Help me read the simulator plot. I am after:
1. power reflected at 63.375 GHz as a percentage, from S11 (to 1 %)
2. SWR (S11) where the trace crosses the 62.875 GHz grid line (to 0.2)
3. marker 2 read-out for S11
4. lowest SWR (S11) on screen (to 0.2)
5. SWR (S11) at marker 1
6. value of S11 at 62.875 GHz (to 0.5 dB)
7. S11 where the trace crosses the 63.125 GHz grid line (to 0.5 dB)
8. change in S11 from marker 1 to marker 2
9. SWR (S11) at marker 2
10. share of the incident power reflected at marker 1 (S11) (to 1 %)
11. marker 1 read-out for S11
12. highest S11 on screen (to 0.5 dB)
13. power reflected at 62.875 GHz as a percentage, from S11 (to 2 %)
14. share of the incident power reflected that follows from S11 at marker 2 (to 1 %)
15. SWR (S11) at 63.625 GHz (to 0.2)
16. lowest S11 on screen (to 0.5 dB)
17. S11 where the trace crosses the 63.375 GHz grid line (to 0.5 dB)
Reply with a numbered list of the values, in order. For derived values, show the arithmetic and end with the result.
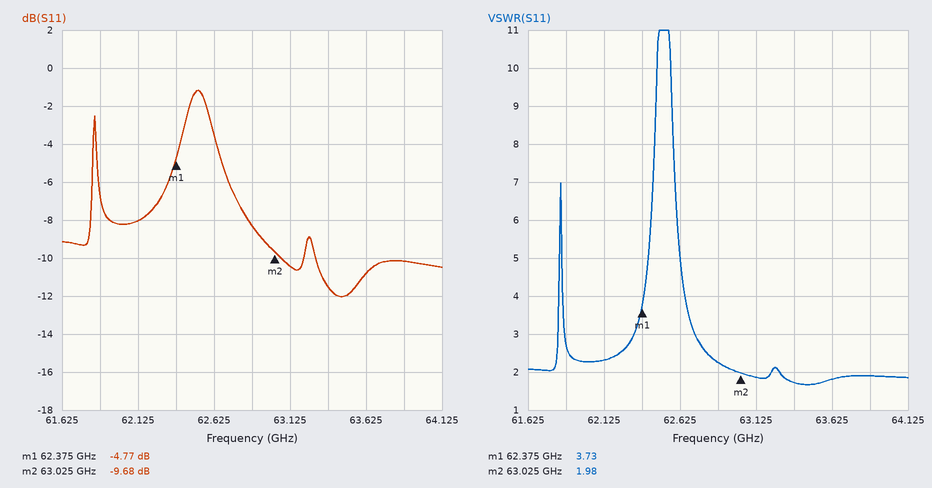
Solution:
1. 10^(-11.5/10) ≈ 7 %
2. 2.2
3. -9.68 dB
4. 1.6
5. 3.73
6. -8.5 dB
7. -10.5 dB
8. -9.68 − (-4.77) = -4.91 dB
9. 1.98
10. 10^(-4.77/10) ≈ 33 %
11. -4.77 dB
12. -1.0 dB
13. 10^(-8.5/10) ≈ 14 %
14. 10^(-9.68/10) ≈ 11 %
15. 1.8
16. -12.0 dB
17. -11.5 dB
